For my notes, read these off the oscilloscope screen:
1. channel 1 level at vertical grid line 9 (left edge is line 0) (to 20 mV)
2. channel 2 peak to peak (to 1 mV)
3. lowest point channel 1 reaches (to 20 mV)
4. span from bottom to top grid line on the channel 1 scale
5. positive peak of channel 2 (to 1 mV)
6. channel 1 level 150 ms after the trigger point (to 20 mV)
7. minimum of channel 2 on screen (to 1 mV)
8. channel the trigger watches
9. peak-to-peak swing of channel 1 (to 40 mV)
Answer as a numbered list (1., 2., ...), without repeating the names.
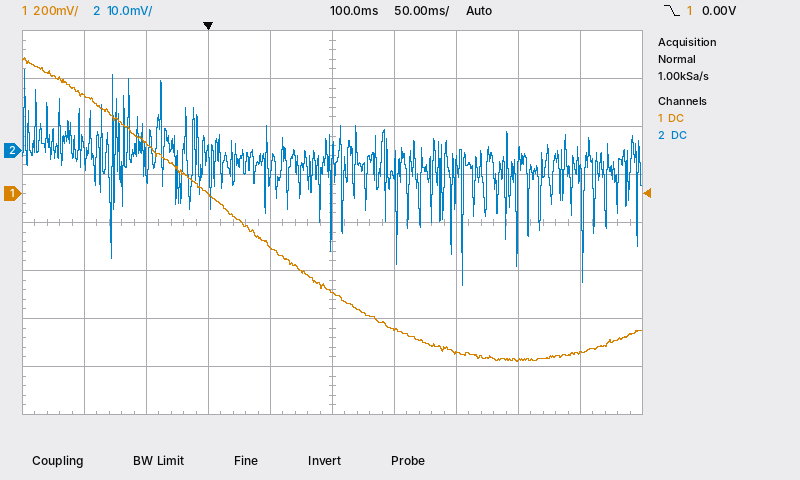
1. -660 mV
2. 45 mV
3. -700 mV
4. 1.6 V
5. 17 mV
6. -560 mV
7. -28 mV
8. channel 1
9. 1.28 V
